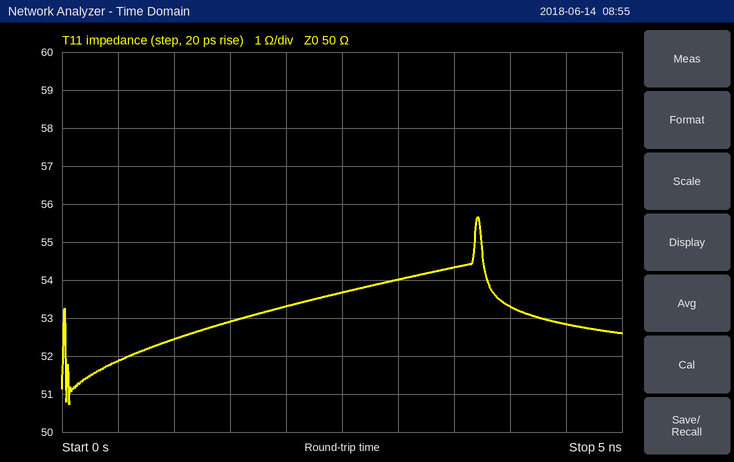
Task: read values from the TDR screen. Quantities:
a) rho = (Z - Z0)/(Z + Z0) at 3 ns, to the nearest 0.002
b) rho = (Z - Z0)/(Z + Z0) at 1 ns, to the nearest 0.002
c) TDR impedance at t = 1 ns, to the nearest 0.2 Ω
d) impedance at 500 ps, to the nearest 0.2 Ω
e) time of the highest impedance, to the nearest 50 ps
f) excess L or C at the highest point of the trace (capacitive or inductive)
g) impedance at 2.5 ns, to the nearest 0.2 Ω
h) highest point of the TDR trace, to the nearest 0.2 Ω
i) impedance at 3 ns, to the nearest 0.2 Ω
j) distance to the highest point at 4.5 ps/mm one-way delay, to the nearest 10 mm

+0.038
+0.024
52.4 Ω
51.8 Ω
3.70 ns
inductive
53.6 Ω
55.6 Ω
54.0 Ω
410 mm
